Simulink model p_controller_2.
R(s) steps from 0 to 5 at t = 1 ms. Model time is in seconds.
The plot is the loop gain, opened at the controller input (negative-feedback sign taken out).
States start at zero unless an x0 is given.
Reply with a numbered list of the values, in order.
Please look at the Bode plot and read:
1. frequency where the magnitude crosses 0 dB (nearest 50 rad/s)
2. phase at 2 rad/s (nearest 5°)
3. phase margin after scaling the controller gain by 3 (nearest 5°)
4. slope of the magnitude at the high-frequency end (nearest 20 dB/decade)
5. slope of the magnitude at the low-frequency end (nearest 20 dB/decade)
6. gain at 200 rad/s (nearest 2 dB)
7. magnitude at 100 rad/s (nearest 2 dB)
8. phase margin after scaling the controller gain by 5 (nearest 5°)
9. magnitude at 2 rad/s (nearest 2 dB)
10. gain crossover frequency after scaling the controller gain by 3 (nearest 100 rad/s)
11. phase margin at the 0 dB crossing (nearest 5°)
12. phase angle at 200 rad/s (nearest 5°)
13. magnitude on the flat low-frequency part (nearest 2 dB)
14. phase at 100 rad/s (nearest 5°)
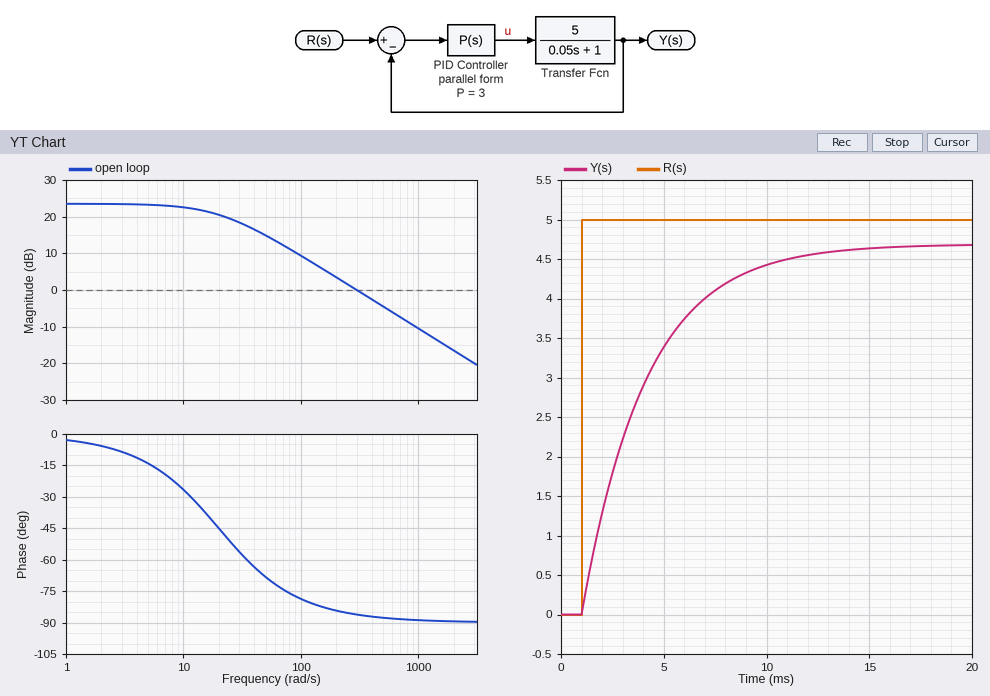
1. 300 rad/s
2. -5°
3. 90°
4. -20 dB/decade
5. 0 dB/decade
6. 4 dB
7. 10 dB
8. 90°
9. 24 dB
10. 900 rad/s
11. 95°
12. -85°
13. 24 dB
14. -80°
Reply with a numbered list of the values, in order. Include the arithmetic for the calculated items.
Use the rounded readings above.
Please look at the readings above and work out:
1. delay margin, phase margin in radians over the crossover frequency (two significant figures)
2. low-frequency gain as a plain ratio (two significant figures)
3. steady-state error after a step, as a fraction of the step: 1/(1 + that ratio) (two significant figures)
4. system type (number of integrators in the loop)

1. 95 × π / 180 / 300 = 0.0055 s
2. 10^(24 / 20) = 16
3. 1 / (1 + 16) = 0.059
4. 0
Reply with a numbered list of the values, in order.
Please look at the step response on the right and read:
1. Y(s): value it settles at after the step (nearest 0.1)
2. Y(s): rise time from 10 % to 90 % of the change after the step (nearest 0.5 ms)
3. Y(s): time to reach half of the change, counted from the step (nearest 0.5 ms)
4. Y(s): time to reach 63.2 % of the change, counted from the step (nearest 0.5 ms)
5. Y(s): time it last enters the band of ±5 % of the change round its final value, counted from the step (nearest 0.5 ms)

1. 4.7
2. 7.0 ms
3. 2.0 ms
4. 3.0 ms
5. 9.5 ms
